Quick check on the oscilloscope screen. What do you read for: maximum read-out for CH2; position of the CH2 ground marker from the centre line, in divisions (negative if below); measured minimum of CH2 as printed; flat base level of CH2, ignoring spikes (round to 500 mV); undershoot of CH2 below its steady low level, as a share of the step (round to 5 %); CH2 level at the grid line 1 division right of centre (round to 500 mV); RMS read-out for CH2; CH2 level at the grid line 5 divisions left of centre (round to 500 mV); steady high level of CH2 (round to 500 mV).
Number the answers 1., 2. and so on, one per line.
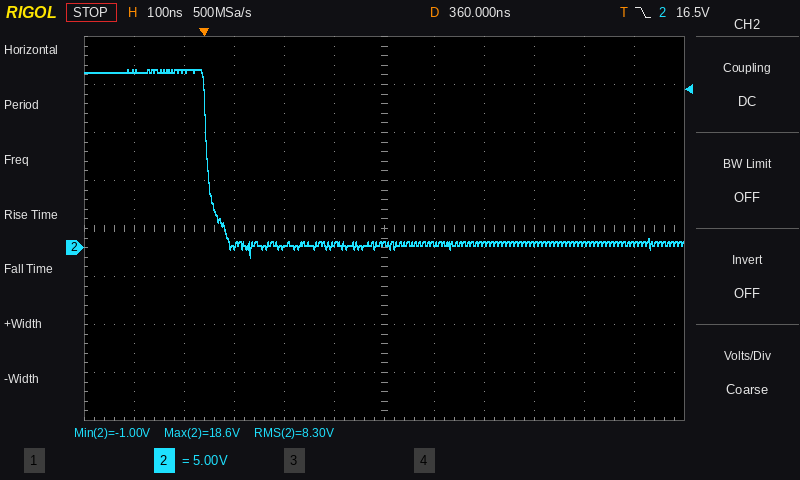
1. 18.6 V
2. -0.4 div
3. -1.00 V
4. 500 mV
5. 10 %
6. 500 mV
7. 8.30 V
8. 18.5 V
9. 18.0 V
